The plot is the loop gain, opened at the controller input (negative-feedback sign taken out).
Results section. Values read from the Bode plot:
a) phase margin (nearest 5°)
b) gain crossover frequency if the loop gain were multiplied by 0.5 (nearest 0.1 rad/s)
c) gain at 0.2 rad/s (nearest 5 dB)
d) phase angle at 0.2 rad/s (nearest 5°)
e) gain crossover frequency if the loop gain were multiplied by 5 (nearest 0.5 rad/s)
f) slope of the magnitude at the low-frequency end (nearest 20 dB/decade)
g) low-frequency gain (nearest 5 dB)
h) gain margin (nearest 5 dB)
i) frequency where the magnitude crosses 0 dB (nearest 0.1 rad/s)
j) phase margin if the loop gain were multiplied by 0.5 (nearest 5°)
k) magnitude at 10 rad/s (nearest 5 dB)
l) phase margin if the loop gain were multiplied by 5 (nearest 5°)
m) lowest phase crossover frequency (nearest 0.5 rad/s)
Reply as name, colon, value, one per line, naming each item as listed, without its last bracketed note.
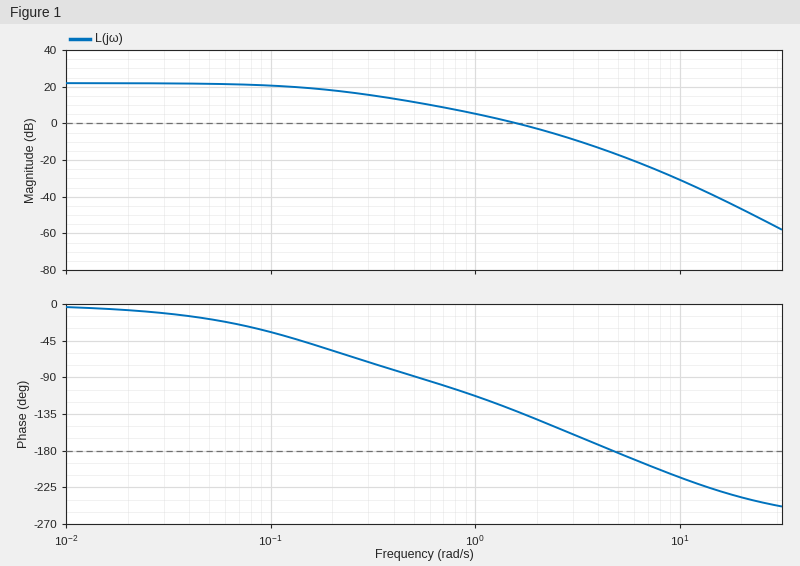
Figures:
phase margin: 50°
gain crossover frequency if the loop gain were multiplied by 0.5: 0.9 rad/s
gain at 0.2 rad/s: 20 dB
phase angle at 0.2 rad/s: -55°
gain crossover frequency if the loop gain were multiplied by 5: 4.0 rad/s
slope of the magnitude at the low-frequency end: 0 dB/decade
low-frequency gain: 20 dB
gain margin: 15 dB
frequency where the magnitude crosses 0 dB: 1.6 rad/s
phase margin if the loop gain were multiplied by 0.5: 70°
magnitude at 10 rad/s: -30 dB
phase margin if the loop gain were multiplied by 5: 5°
lowest phase crossover frequency: 4.5 rad/s
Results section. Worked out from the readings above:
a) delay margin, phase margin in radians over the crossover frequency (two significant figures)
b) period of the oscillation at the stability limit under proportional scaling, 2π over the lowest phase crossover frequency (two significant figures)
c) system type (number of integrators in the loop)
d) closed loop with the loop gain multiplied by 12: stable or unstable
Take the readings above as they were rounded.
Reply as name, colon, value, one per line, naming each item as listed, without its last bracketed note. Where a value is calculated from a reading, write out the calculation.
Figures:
delay margin, phase margin in radians over the crossover frequency: 50 × π / 180 / 1.6 = 0.55 s
period of the oscillation at the stability limit under proportional scaling, 2π over the lowest phase crossover frequency: 2π / 4.5 = 1.4 s
system type: 0
closed loop with the loop gain multiplied by 12: stable or unstable: unstable
